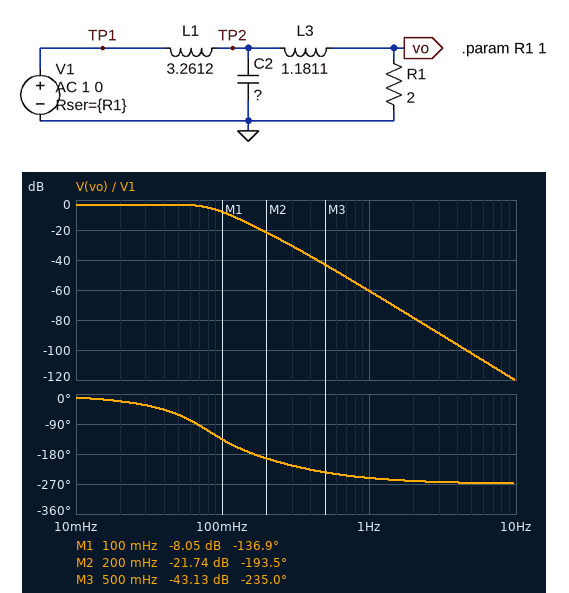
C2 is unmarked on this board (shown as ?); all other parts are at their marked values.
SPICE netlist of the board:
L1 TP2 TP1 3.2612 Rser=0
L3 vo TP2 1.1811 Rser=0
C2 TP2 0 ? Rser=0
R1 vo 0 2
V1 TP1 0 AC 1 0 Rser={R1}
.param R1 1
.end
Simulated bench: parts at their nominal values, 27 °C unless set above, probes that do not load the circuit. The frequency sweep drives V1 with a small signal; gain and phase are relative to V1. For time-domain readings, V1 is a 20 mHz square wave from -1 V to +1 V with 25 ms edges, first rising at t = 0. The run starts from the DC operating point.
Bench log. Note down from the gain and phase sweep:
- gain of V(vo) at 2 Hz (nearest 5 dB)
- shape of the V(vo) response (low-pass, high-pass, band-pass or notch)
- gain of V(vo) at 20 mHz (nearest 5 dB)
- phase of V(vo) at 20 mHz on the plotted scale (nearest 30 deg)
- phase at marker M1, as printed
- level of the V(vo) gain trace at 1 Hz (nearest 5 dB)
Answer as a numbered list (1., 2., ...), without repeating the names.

1. -80 dB
2. low-pass
3. -5 dB
4. -30 deg
5. -136.9 deg
6. -60 dB
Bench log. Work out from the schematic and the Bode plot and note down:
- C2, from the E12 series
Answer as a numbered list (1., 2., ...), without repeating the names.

1. 2.2 F
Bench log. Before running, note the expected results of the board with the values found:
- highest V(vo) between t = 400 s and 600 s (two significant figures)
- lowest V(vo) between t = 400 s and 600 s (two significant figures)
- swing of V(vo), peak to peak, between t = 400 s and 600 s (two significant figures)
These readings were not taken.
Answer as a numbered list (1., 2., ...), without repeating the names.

1. 820 mV
2. -820 mV
3. 1.6 V
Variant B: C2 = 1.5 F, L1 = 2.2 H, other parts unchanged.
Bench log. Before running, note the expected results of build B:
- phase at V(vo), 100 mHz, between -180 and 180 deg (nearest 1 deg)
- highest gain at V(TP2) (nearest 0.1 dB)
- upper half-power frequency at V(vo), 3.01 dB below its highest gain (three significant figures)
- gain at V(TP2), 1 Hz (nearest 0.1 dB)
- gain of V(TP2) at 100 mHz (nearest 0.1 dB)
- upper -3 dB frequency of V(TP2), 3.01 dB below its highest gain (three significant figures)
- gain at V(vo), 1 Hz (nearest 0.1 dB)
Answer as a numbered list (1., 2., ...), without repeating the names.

1. -96 deg
2. -2.7 dB
3. 130 mHz
4. -42.1 dB
5. -3.1 dB
6. 136 mHz
7. -53.8 dB
